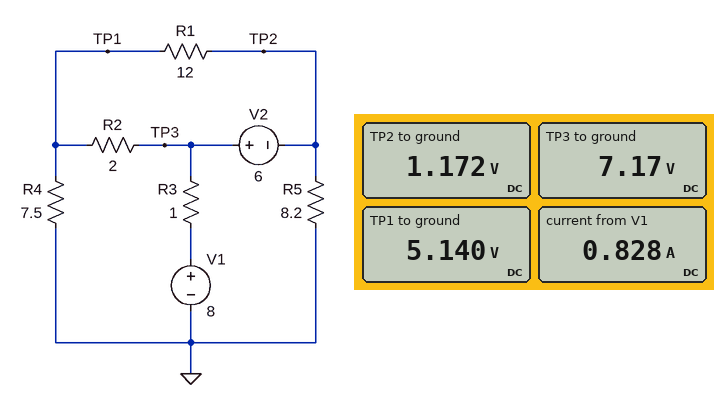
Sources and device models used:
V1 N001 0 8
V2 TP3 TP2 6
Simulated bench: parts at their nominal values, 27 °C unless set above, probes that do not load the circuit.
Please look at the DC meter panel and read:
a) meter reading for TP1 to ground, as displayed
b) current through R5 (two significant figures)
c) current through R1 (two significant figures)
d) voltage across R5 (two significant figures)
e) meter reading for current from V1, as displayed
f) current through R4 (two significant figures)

5.140 V
140 mA
330 mA
1.2 V
0.828 A
690 mA
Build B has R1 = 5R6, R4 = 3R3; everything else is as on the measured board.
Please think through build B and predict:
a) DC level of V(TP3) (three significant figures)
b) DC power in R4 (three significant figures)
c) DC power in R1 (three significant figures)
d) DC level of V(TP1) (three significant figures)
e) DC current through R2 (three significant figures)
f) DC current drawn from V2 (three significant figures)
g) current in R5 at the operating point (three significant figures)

6.81 V
3.96 W
1.41 W
3.61 V
1.60 A
403 mA
98.4 mA
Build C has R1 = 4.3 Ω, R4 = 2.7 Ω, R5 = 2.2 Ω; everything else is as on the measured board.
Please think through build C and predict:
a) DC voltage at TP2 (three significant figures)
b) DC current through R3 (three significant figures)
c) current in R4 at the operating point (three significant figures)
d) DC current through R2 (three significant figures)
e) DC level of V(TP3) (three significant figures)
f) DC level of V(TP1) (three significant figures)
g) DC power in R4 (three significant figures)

584 mV
1.42 A
1.15 A
1.74 A
6.58 V
3.11 V
3.58 W
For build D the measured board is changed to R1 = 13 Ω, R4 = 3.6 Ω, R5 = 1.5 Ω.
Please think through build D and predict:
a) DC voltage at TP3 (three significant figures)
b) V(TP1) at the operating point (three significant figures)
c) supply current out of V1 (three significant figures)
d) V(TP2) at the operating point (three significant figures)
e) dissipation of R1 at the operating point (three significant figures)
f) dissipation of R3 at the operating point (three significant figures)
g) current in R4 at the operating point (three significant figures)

6.55 V
3.88 V
1.45 A
553 mV
853 mW
2.09 W
1.08 A
